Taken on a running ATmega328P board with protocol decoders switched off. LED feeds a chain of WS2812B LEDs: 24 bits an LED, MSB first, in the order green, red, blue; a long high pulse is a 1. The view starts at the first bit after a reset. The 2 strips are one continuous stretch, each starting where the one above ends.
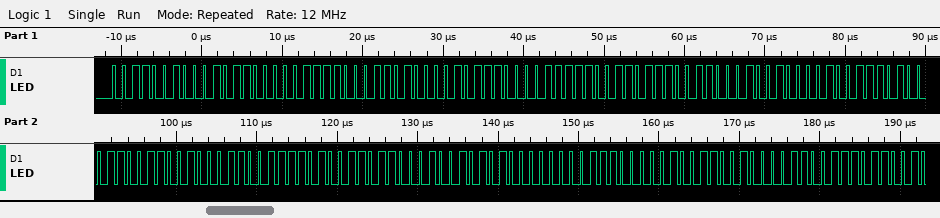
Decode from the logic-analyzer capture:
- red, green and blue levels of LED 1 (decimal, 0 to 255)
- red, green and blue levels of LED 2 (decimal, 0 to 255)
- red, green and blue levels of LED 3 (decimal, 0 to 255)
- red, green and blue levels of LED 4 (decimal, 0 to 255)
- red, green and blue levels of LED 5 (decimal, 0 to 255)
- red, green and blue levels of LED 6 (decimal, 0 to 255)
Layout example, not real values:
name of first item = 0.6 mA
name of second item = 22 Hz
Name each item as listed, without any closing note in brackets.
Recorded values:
red, green and blue levels of LED 1 = 44, 50, 30
red, green and blue levels of LED 2 = 46, 52, 31
red, green and blue levels of LED 3 = 49, 55, 33
red, green and blue levels of LED 4 = 51, 58, 35
red, green and blue levels of LED 5 = 54, 61, 37
red, green and blue levels of LED 6 = 56, 64, 38
